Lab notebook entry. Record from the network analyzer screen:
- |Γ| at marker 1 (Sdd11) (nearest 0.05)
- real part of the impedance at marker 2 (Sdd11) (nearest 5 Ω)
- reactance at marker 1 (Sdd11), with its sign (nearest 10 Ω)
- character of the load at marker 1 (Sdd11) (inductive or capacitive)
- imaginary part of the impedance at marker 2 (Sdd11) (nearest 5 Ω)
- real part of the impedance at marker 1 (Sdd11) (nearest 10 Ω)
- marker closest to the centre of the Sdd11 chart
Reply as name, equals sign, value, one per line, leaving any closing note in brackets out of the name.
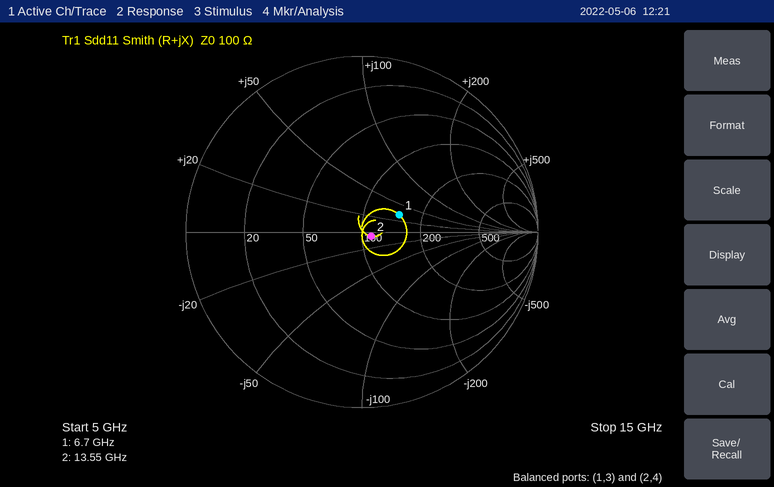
|Γ| at marker 1 (Sdd11) = 0.25
real part of the impedance at marker 2 (Sdd11) = 110 Ω
reactance at marker 1 (Sdd11), with its sign = +30 Ω
character of the load at marker 1 (Sdd11) = inductive
imaginary part of the impedance at marker 2 (Sdd11) = -5 Ω
real part of the impedance at marker 1 (Sdd11) = 150 Ω
marker closest to the centre of the Sdd11 chart = marker 2
